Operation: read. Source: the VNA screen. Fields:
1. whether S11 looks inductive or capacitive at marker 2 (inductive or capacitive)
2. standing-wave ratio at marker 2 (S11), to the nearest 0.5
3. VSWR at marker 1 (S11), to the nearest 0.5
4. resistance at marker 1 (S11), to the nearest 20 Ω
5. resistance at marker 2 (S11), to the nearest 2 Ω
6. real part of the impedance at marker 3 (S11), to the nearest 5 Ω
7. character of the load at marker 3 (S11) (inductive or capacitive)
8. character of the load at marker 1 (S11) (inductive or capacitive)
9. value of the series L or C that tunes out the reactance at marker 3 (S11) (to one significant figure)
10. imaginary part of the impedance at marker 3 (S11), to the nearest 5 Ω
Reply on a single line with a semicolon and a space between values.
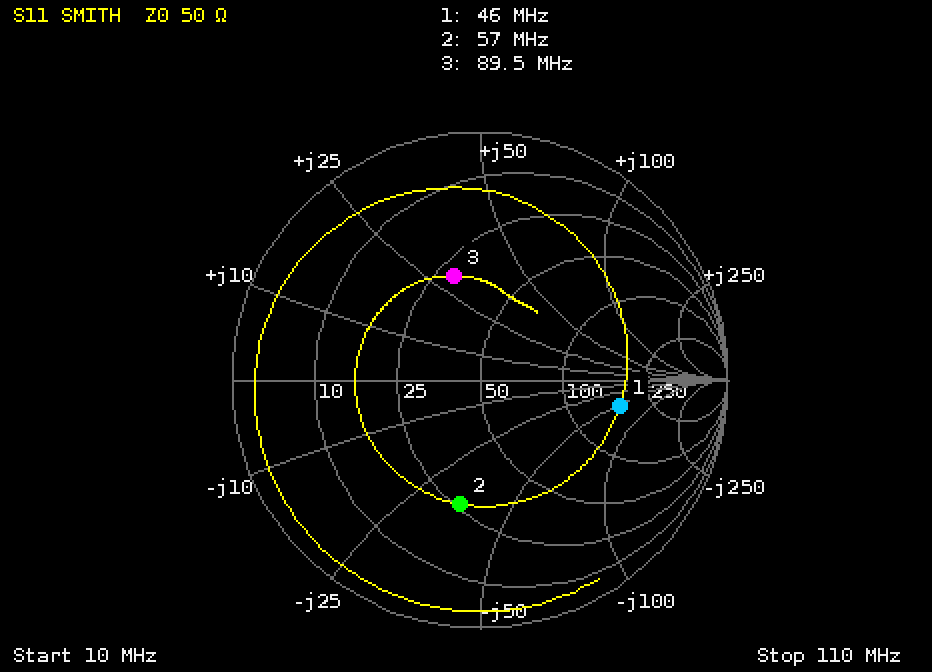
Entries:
capacitive; 3.0; 3.5; 160 Ω; 26 Ω; 30 Ω; inductive; capacitive; 60 pF; +30 Ω
